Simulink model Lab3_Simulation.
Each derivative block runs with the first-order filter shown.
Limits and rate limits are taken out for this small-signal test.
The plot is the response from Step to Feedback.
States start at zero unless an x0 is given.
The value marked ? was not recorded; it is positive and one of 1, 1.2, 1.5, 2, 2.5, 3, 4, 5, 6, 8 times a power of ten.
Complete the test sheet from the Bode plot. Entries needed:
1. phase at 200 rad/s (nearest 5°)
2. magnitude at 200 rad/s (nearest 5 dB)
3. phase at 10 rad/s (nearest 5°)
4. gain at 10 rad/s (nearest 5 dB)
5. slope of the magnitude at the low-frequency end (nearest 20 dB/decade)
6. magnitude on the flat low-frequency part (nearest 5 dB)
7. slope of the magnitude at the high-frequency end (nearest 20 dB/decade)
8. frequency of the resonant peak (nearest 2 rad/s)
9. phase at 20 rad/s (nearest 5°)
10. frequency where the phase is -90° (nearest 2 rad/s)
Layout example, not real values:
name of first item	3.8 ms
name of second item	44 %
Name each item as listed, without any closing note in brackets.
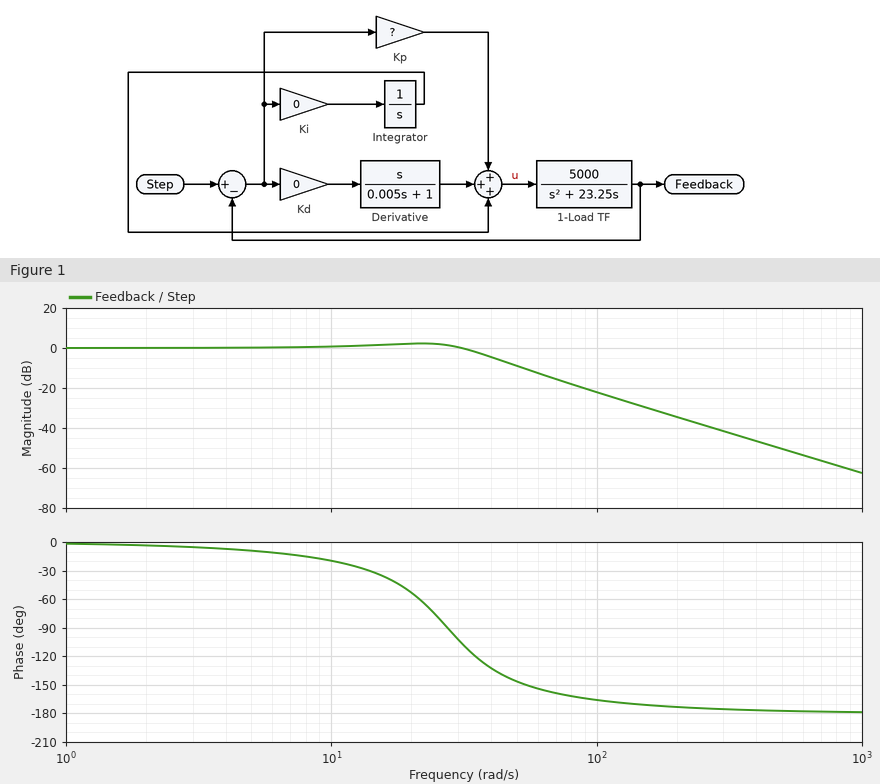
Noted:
phase at 200 rad/s	-175°
magnitude at 200 rad/s	-35 dB
phase at 10 rad/s	-20°
gain at 10 rad/s	0 dB
slope of the magnitude at the low-frequency end	0 dB/decade
magnitude on the flat low-frequency part	0 dB
slope of the magnitude at the high-frequency end	-40 dB/decade
frequency of the resonant peak	22 rad/s
phase at 20 rad/s	-55°
frequency where the phase is -90°	28 rad/s
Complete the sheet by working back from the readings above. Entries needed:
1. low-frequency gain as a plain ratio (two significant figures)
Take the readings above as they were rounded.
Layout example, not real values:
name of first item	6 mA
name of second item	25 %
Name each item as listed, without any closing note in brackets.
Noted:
low-frequency gain as a plain ratio	1.0
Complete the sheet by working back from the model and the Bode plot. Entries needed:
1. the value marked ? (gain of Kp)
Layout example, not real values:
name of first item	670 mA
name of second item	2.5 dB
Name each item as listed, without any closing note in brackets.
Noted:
the value marked ?	0.15
